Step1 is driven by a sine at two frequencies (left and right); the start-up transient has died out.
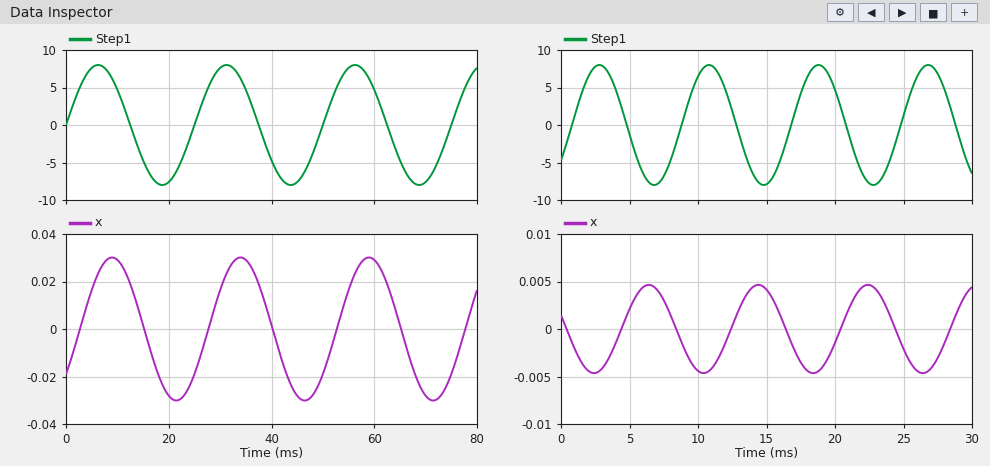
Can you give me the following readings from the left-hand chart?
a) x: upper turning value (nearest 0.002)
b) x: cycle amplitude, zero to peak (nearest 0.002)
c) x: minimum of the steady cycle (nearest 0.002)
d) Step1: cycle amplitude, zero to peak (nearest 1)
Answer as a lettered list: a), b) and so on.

a) 0.030
b) 0.030
c) -0.030
d) 8
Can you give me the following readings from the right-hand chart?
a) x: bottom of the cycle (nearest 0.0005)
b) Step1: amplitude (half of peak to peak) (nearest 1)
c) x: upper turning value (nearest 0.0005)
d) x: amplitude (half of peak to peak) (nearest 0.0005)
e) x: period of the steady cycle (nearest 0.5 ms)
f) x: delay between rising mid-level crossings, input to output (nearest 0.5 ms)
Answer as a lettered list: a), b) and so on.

a) -0.0045
b) 8
c) 0.0045
d) 0.0045
e) 8.0 ms
f) 3.5 ms
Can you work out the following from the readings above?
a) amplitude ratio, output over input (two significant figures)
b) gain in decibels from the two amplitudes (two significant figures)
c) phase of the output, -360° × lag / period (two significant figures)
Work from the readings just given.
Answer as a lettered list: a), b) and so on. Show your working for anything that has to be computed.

a) 0.0045 / 8 = 0.00056
b) 20 log10(0.0045 / 8) = -65 dB
c) -360 × 3.5 / 8 = -160°
